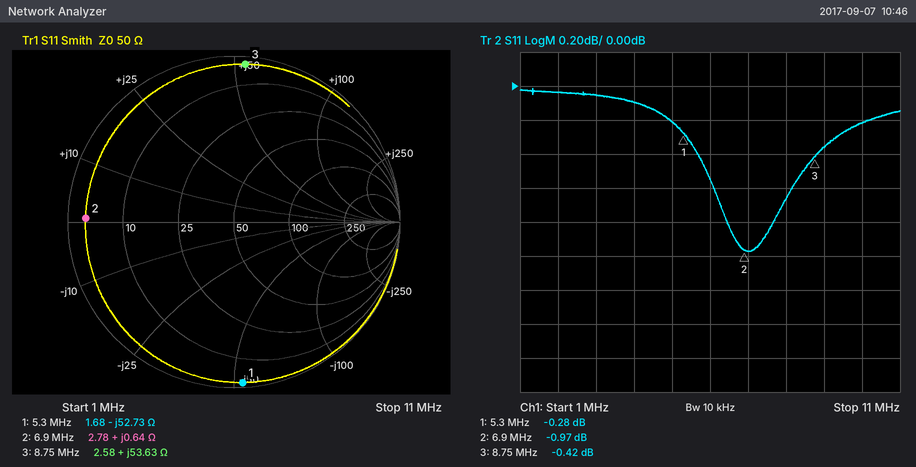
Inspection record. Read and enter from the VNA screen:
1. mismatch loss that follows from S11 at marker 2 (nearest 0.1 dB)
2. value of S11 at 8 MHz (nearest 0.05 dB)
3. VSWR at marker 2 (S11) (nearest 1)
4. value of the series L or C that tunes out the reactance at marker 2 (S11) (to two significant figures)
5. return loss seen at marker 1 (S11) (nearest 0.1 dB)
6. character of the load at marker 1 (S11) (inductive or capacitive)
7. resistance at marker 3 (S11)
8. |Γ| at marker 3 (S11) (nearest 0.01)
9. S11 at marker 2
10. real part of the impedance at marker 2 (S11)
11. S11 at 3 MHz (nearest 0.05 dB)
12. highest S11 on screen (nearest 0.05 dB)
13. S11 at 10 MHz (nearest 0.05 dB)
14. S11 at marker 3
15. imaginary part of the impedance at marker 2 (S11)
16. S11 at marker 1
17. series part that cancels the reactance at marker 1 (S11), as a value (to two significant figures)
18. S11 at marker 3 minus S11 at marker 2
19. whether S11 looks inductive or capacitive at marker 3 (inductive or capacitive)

7.0 dB
-0.65 dB
18
36 nF
0.3 dB
capacitive
2.58 Ω
0.95
-0.97 dB
2.78 Ω
-0.05 dB
0.00 dB
-0.20 dB
-0.42 dB
+0.64 Ω
-0.28 dB
1.6 µH
0.55 dB
inductive
